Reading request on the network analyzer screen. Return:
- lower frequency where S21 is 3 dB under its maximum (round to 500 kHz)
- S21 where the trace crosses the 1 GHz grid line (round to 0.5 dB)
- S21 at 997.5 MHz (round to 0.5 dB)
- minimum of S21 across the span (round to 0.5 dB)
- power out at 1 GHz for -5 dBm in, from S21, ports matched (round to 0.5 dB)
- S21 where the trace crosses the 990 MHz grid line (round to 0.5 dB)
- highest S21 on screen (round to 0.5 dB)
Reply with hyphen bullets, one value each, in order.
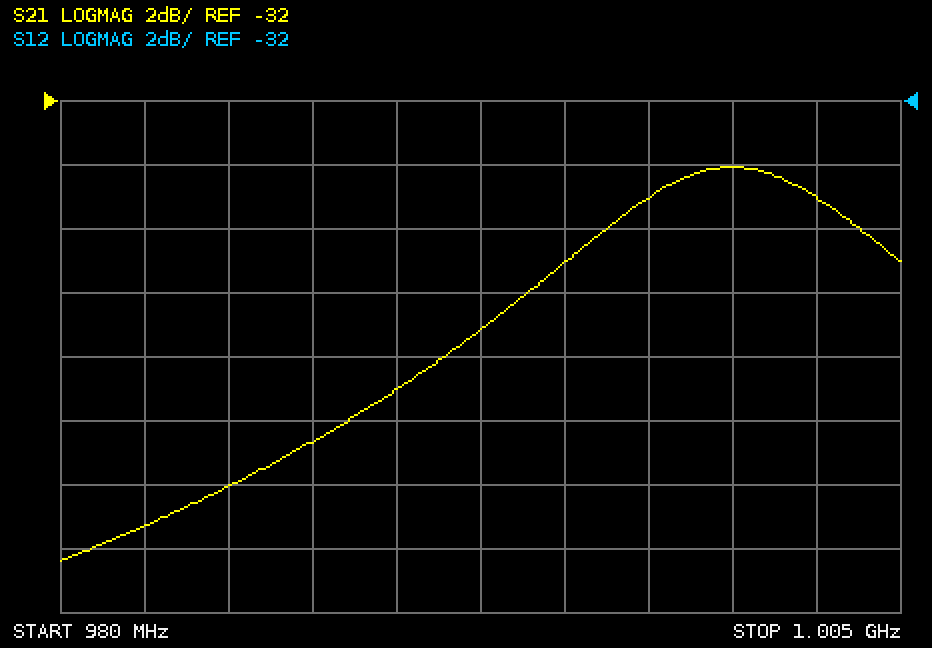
- 995.0 MHz
- -34.0 dB
- -35.0 dB
- -46.5 dB
- -39.0 dBm
- -41.0 dB
- -34.0 dB
